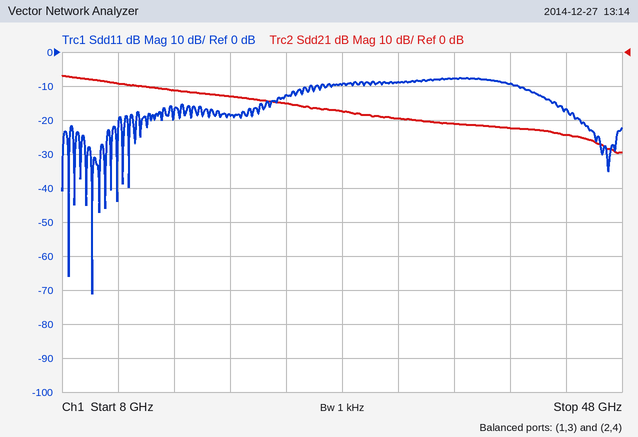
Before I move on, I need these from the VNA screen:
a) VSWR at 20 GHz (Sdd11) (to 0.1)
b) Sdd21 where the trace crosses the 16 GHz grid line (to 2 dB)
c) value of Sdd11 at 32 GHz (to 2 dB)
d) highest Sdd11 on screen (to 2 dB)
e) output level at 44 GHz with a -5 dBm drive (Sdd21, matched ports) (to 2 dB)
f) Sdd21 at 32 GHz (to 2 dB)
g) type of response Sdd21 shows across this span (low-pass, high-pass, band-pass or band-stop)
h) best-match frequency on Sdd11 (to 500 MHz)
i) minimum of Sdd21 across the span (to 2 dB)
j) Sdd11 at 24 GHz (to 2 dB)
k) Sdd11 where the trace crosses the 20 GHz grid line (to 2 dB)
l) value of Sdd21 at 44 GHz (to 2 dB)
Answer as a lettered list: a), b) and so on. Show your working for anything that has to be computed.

a) |Γ| = 10^(-18/20) = 0.1259; VSWR = (1 + 0.1259)/(1 − 0.1259) ≈ 1.3
b) -12 dB
c) -8 dB
d) -8 dB
e) -5 dBm + (-24 dB) = -30 dBm
f) -20 dB
g) low-pass
h) 10.0 GHz
i) -30 dB
j) -12 dB
k) -18 dB
l) -24 dB
